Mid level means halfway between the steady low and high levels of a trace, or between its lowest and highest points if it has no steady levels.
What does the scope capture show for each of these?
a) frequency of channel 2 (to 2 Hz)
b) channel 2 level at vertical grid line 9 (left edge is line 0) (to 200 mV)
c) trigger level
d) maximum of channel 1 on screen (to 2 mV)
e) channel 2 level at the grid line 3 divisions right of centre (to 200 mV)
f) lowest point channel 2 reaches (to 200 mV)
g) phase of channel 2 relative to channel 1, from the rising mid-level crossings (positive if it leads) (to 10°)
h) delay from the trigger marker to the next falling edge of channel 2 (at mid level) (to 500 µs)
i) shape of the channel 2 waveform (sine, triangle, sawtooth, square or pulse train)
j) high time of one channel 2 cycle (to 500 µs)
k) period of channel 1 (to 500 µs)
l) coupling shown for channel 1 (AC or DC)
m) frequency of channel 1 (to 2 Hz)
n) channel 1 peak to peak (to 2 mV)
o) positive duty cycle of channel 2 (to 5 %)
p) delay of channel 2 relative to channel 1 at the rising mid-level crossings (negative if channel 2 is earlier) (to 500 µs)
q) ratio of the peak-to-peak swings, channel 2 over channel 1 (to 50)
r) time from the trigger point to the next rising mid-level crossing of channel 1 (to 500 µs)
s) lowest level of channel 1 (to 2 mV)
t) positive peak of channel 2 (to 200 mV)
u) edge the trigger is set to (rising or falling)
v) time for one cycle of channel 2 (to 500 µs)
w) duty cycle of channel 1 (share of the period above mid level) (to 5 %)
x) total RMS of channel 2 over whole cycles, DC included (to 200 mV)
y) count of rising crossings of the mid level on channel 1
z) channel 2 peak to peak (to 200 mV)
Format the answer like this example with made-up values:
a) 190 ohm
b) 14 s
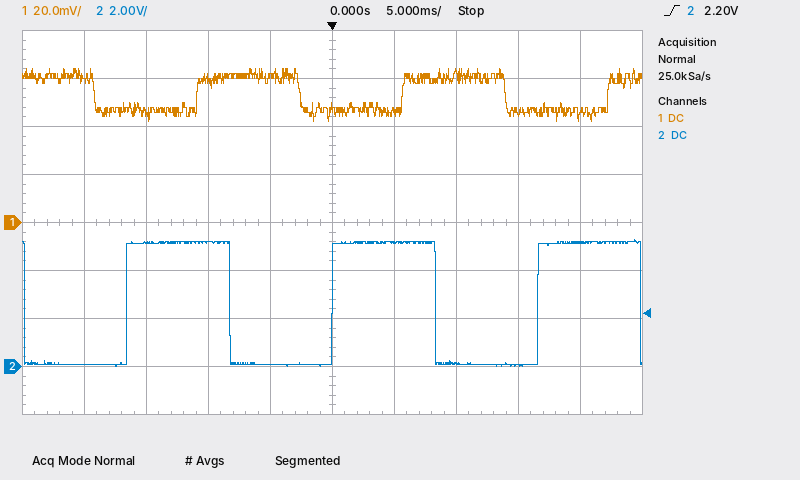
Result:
a) 60 Hz
b) 5.2 V
c) 2.20 V
d) 64 mV
e) 0.0 V
f) 0.0 V
g) +120°
h) 8.5 ms
i) square
j) 8.5 ms
k) 16.5 ms
l) DC
m) 60 Hz
n) 22 mV
o) 50 %
p) -5.5 ms
q) 250
r) 5.5 ms
s) 42 mV
t) 5.2 V
u) rising
v) 16.5 ms
w) 50 %
x) 3.6 V
y) 3
z) 5.2 V
